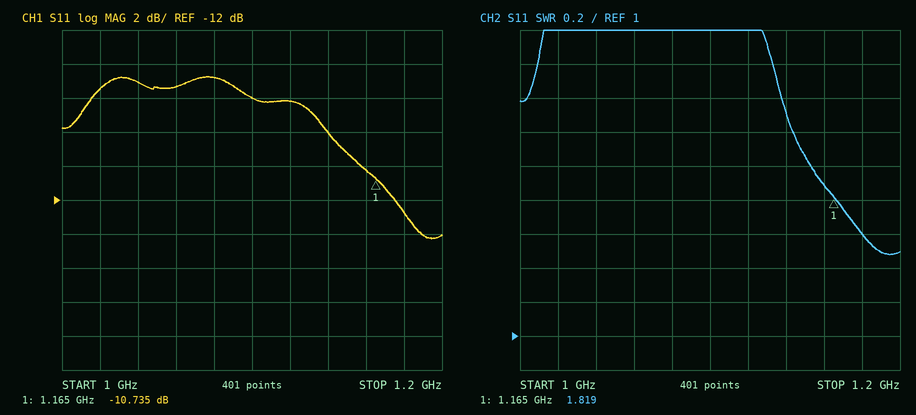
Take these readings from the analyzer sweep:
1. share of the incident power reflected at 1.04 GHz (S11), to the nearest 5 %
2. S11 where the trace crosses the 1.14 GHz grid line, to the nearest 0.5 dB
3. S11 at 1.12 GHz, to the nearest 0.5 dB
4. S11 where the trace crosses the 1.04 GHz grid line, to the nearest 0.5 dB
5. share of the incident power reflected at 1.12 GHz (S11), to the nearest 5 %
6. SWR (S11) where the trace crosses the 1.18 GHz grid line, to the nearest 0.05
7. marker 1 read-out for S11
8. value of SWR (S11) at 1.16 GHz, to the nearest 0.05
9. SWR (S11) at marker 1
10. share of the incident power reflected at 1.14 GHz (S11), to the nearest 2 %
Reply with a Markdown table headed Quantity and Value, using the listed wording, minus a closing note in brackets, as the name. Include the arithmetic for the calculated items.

| Quantity | Value |
|---|---|
| share of the incident power reflected at 1.04 GHz (S11), to the nearest 5 % | 10^(-5/10) ≈ 31.6 %, so 30 % to the nearest 5 % |
| S11 where the trace crosses the 1.14 GHz grid line, to the nearest 0.5 dB | -8.0 dB |
| S11 at 1.12 GHz, to the nearest 0.5 dB | -6.0 dB |
| S11 where the trace crosses the 1.04 GHz grid line, to the nearest 0.5 dB | -5.0 dB |
| share of the incident power reflected at 1.12 GHz (S11), to the nearest 5 % | 10^(-6/10) ≈ 25 % |
| SWR (S11) where the trace crosses the 1.18 GHz grid line, to the nearest 0.05 | 1.60 |
| marker 1 read-out for S11 | -10.735 dB |
| value of SWR (S11) at 1.16 GHz, to the nearest 0.05 | 1.90 |
| SWR (S11) at marker 1 | 1.819 |
| share of the incident power reflected at 1.14 GHz (S11), to the nearest 2 % | 10^(-8/10) ≈ 16 % |
